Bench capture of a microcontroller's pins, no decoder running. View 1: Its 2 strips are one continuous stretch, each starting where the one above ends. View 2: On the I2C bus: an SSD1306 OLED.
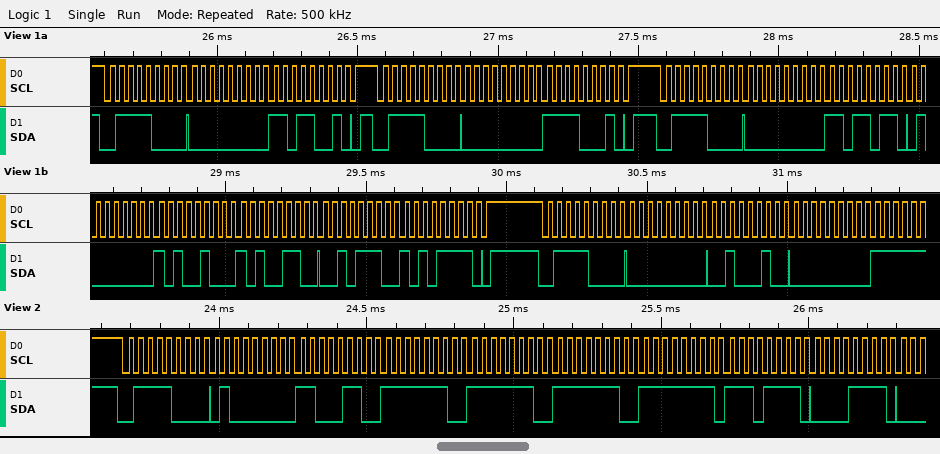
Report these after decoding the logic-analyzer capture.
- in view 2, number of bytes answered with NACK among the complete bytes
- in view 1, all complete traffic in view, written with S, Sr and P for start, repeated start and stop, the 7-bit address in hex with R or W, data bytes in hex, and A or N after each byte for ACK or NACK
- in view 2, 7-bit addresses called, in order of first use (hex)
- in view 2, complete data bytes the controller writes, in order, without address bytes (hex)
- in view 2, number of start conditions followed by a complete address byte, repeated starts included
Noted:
0
S 3CW A 00 A D9 A P S 3CW A 00 A F1 A P S 3CW A 00 A DB A 40 A A4 A A6 A 2E A AF A P S 3CW A 00 A 22 A 00 A
0x3C
40 C6 FE FE FE FF EF 0F
1
